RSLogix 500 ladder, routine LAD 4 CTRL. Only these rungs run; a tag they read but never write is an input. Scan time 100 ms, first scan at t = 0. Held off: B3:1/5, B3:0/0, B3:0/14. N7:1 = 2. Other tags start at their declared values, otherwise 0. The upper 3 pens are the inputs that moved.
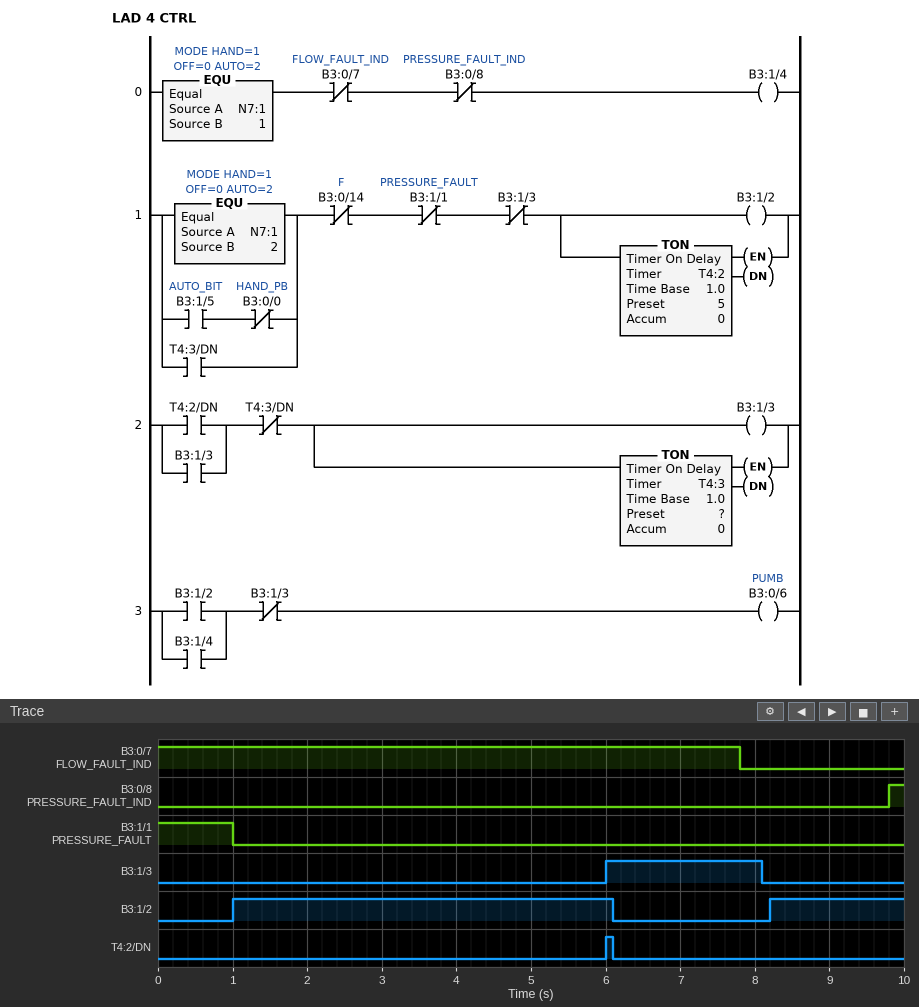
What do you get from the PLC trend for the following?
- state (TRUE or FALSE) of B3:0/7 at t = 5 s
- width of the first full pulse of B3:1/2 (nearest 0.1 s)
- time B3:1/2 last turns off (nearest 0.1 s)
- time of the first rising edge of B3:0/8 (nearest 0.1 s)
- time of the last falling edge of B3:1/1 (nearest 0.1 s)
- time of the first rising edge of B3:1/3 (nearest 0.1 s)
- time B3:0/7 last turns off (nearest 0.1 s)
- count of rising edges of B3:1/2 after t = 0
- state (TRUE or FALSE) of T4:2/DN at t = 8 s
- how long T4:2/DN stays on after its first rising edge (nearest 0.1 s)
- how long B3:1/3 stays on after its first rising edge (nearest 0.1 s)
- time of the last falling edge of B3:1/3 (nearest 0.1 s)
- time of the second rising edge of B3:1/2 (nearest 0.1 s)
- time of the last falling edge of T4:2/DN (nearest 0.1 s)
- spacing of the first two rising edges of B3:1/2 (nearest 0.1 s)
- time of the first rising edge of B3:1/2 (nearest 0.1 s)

TRUE
5.1 s
6.1 s
9.8 s
1.0 s
6.0 s
7.8 s
2
FALSE
0.1 s
2.1 s
8.1 s
8.2 s
6.1 s
7.2 s
1.0 s
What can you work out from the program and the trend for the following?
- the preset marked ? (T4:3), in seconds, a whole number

2 s
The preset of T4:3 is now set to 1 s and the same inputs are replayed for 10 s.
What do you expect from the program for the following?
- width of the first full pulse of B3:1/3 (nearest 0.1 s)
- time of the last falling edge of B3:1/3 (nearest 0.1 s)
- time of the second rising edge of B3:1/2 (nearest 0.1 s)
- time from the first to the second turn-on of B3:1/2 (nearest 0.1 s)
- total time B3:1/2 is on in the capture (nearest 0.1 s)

1.1 s
7.1 s
7.2 s
6.2 s
7.9 s
